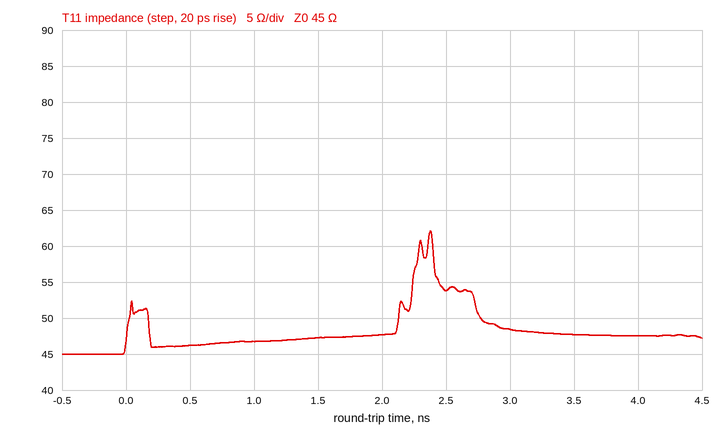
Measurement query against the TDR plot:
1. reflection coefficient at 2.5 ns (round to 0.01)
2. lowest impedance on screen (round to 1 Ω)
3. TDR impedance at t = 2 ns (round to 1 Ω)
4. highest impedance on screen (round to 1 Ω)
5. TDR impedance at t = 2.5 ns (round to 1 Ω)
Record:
+0.09
45 Ω
48 Ω
62 Ω
54 Ω
